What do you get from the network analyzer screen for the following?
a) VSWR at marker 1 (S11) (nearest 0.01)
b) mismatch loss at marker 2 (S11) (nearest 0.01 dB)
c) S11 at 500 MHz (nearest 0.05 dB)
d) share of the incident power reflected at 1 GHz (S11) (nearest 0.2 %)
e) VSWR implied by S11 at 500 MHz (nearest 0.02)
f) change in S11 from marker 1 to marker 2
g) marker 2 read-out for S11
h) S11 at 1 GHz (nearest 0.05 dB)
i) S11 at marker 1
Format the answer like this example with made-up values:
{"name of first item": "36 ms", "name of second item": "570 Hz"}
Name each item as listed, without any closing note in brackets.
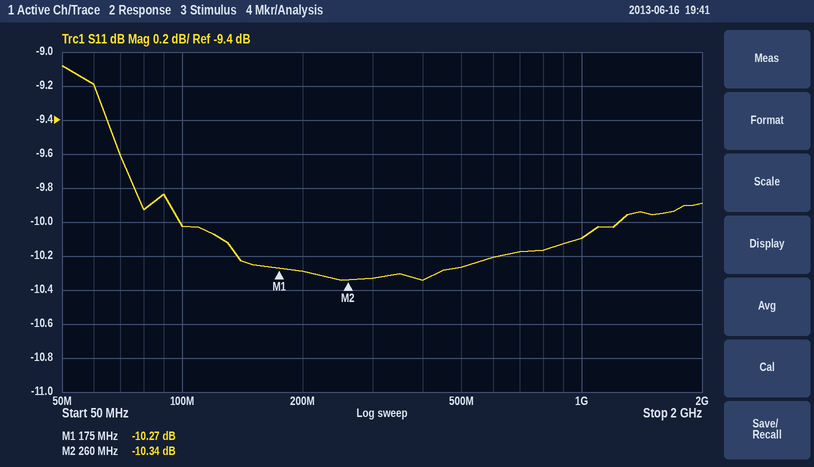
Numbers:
{"VSWR at marker 1 (S11)": "1.88", "mismatch loss at marker 2 (S11)": "0.42 dB", "S11 at 500 MHz": "-10.25 dB", "share of the incident power reflected at 1 GHz (S11)": "9.8 %", "VSWR implied by S11 at 500 MHz": "1.88", "change in S11 from marker 1 to marker 2": "-0.07 dB", "marker 2 read-out for S11": "-10.34 dB", "S11 at 1 GHz": "-10.10 dB", "S11 at marker 1": "-10.27 dB"}
